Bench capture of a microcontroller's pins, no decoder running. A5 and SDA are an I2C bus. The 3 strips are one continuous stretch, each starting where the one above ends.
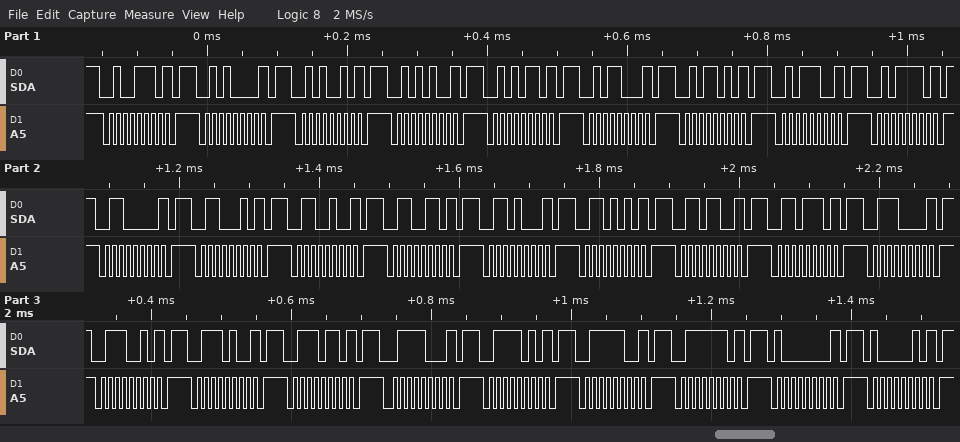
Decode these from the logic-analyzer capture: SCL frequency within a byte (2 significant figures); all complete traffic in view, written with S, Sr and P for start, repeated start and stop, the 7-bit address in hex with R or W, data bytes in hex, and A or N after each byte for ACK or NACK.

100 kHz
S 27W N P S 28W N P S 29W N P S 2AW N P S 2BW N P S 2CW N P S 2DW N P S 2EW N P S 2FW N P S 30W N P S 31W N P S 32W N P S 33W N P S 34W N P S 35W N P S 36W N P S 37W N P S 38W N P S 39W N P S 3AW N P S 3BW N P S 3CW N P S 3DW N P S 3EW N P S 3FW N P S 40W N P S 41W N P
